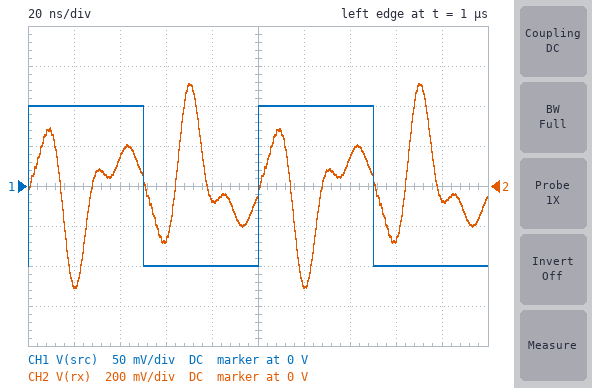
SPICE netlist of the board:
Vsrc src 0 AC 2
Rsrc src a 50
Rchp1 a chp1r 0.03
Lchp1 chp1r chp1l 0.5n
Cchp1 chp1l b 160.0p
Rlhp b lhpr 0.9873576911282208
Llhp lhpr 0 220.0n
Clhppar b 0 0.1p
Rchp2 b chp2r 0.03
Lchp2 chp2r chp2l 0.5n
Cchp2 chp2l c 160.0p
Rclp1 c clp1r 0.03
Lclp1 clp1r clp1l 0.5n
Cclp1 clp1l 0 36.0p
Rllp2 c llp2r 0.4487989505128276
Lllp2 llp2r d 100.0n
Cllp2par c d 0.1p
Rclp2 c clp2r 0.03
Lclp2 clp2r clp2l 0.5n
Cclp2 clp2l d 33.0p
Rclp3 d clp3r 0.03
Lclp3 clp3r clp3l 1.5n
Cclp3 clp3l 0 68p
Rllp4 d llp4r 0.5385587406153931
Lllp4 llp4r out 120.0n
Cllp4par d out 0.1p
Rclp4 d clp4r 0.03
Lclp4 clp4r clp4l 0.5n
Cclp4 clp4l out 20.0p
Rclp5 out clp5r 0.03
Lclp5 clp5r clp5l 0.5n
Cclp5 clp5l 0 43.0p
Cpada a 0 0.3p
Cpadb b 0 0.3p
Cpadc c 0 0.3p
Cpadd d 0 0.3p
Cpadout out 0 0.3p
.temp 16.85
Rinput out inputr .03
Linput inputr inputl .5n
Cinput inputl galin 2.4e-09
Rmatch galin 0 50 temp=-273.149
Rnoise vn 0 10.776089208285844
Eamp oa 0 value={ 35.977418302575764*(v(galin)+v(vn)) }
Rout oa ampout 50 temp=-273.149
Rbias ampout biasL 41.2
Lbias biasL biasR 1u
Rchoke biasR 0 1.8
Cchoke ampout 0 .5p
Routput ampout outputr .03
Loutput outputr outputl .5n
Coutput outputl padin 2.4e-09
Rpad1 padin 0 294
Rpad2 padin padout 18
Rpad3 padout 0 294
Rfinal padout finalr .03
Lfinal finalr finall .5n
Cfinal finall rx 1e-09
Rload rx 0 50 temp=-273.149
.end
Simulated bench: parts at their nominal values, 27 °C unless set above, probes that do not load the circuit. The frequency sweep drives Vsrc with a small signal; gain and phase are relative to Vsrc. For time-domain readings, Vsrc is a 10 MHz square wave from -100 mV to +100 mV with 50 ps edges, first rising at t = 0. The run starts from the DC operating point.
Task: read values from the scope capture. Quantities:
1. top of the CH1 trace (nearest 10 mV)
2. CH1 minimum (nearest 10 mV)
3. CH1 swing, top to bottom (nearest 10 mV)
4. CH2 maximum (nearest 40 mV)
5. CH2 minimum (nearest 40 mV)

100 mV
-100 mV
200 mV
520 mV
-520 mV
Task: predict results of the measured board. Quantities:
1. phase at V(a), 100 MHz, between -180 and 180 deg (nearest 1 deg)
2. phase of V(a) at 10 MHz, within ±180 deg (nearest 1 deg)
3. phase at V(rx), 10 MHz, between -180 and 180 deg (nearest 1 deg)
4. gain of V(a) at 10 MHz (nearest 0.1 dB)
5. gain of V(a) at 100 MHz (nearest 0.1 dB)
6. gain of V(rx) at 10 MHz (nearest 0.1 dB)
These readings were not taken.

-33 deg
-30 deg
-147 deg
-1.4 dB
-1.6 dB
-4.1 dB
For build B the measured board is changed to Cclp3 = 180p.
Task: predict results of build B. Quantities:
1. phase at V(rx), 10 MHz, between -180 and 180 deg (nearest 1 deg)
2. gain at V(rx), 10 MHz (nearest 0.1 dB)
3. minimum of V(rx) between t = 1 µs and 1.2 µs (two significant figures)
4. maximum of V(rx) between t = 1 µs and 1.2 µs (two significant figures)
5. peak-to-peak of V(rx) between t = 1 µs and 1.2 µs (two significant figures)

-155 deg
-5.5 dB
-400 mV
400 mV
810 mV
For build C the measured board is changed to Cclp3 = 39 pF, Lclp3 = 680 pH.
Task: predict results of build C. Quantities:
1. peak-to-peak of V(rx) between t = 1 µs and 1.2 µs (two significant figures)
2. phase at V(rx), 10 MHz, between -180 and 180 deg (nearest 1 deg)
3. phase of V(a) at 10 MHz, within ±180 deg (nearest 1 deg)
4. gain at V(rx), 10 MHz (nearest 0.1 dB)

990 mV
-145 deg
-30 deg
-3.7 dB
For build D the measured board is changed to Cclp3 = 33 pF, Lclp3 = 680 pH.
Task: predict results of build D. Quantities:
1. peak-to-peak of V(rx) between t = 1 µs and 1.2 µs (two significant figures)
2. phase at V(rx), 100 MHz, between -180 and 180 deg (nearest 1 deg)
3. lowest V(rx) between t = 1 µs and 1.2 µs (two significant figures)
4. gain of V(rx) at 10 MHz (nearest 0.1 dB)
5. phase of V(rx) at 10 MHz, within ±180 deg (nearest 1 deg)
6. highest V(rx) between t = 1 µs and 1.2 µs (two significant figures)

940 mV
-164 deg
-470 mV
-3.6 dB
-144 deg
470 mV
